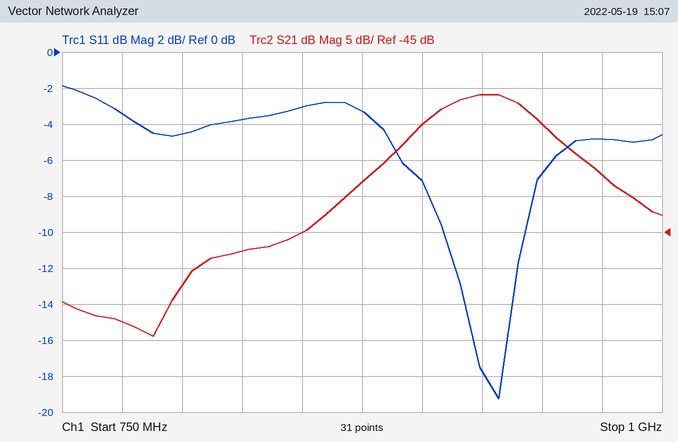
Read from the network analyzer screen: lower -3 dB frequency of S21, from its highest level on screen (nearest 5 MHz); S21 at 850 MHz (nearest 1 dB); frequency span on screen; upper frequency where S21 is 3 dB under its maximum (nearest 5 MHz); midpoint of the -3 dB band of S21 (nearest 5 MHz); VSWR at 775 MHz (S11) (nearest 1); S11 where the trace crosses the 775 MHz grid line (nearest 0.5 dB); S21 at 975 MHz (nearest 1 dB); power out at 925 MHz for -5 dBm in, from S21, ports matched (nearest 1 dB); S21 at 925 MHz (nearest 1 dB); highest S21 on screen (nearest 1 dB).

905 MHz
-45 dB
250 MHz
945 MHz
925 MHz
5
-3.5 dB
-37 dB
-31 dBm
-26 dB
-26 dB
